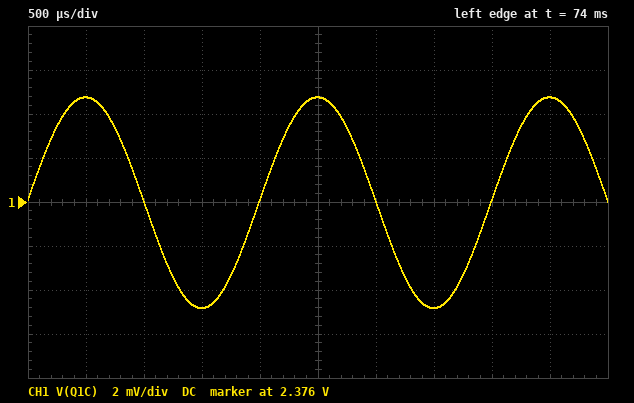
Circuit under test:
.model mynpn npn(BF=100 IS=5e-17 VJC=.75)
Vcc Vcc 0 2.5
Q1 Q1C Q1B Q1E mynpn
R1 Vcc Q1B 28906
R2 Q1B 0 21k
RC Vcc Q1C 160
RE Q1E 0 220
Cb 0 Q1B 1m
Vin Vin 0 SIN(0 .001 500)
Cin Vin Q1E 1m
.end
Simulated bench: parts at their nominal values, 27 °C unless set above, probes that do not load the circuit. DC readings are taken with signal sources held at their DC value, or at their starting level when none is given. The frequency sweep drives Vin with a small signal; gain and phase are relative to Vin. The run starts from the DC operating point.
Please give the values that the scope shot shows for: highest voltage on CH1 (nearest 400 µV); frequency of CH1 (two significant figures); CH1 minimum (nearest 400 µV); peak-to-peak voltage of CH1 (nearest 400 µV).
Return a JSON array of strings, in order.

["2.3808 V", "500 Hz", "2.3712 V", "9.6 mV"]
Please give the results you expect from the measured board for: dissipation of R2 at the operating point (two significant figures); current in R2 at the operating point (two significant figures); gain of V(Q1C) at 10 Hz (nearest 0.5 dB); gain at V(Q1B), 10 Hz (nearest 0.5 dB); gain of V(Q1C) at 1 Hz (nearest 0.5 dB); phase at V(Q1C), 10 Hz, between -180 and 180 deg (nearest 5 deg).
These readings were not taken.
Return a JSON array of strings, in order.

["44 µW", "46 µA", "12.5 dB", "-47.5 dB", "-1.5 dB", "30 deg"]
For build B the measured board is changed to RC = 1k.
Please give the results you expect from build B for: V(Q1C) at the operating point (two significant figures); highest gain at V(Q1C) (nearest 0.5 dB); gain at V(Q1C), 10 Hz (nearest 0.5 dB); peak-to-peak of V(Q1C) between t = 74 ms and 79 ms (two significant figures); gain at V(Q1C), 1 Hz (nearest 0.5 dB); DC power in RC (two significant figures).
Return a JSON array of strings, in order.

["1.7 V", "29.5 dB", "28.5 dB", "60 mV", "14.5 dB", "600 µW"]
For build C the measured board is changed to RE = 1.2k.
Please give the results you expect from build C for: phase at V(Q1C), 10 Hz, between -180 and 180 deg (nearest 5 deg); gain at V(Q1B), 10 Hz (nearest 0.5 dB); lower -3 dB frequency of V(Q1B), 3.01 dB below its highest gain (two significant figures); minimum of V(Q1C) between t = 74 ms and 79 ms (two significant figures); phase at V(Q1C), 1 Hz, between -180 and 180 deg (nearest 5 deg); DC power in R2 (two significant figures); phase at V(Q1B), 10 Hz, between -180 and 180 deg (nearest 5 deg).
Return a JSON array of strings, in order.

["10 deg", "-57.5 dB", "14 mHz", "2.5 V", "55 deg", "50 µW", "-80 deg"]
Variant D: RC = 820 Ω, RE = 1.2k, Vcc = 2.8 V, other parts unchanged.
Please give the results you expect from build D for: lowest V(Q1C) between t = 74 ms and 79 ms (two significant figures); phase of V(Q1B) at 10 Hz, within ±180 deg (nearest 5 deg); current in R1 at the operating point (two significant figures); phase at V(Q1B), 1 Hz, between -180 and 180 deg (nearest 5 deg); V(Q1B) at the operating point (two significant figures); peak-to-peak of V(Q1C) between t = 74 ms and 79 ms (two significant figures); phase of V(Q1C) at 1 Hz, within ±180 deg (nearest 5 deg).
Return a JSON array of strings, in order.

["2.5 V", "-80 deg", "57 µA", "-25 deg", "1.1 V", "20 mV", "65 deg"]
